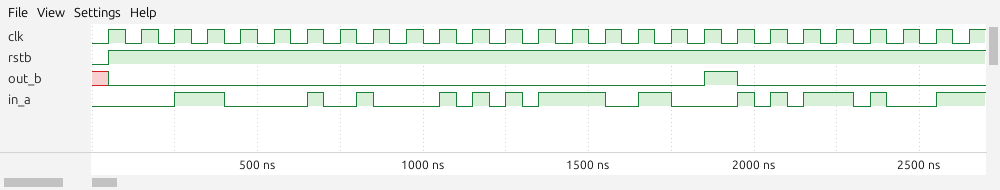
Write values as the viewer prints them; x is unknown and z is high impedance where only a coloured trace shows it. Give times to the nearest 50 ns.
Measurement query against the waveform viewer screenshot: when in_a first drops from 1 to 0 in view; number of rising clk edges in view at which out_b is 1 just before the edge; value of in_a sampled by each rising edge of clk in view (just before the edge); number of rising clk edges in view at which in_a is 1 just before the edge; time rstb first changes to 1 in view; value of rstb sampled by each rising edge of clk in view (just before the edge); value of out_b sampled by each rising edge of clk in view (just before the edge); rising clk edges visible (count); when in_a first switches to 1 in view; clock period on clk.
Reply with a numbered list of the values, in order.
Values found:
1. 400 ns
2. 1
3. 0 0 0 1 0 0 0 0 1 0 0 0 0 0 1 1 0 1 0 0 0 0 1 0 0 0 1
4. 7
5. 50 ns
6. 0 1 1 1 1 1 1 1 1 1 1 1 1 1 1 1 1 1 1 1 1 1 1 1 1 1 1
7. x 0 0 0 0 0 0 0 0 0 0 0 0 0 0 0 0 0 0 1 0 0 0 0 0 0 0
8. 27
9. 250 ns
10. 100 ns
